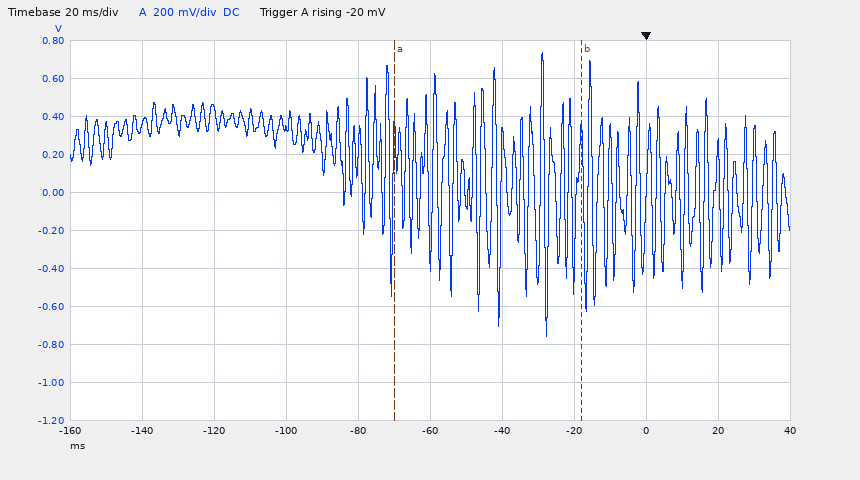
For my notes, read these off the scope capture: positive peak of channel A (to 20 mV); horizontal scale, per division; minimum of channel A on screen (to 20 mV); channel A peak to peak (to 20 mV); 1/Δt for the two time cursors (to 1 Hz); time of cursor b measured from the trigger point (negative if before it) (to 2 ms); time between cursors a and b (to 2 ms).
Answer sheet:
740 mV
20 ms
-760 mV
1.50 V
19 Hz
-18 ms
52 ms
